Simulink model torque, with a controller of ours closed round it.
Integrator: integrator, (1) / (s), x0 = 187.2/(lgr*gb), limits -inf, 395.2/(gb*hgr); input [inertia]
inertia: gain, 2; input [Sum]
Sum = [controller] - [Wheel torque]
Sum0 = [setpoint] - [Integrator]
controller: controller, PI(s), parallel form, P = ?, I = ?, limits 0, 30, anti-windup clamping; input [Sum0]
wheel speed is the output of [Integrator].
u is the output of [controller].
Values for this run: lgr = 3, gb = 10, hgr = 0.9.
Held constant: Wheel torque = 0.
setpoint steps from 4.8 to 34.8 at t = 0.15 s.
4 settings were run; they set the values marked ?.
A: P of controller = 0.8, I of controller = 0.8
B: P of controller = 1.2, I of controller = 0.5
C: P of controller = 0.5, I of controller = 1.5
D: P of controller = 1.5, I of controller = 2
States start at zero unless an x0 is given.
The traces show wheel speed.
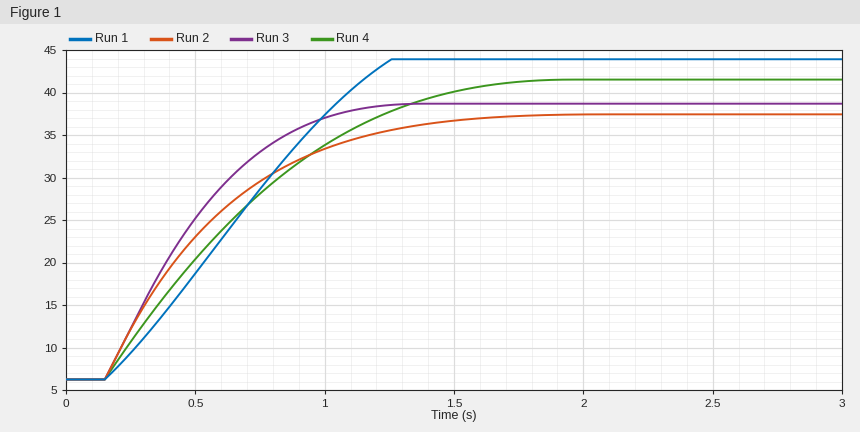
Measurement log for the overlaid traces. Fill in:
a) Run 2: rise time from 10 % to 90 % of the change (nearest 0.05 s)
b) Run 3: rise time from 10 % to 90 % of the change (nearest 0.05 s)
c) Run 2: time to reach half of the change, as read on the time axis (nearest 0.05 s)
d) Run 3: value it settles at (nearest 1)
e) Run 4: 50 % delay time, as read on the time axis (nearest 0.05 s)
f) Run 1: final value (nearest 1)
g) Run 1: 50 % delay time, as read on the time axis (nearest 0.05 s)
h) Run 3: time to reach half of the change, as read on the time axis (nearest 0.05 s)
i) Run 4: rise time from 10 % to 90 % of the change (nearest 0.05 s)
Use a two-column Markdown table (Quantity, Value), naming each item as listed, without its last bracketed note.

| Quantity | Value |
|---|---|
| Run 2: rise time from 10 % to 90 % of the change | 0.90 s |
| Run 3: rise time from 10 % to 90 % of the change | 0.65 s |
| Run 2: time to reach half of the change, as read on the time axis | 0.45 s |
| Run 3: value it settles at | 39 |
| Run 4: 50 % delay time, as read on the time axis | 0.60 s |
| Run 1: final value | 44 |
| Run 1: 50 % delay time, as read on the time axis | 0.65 s |
| Run 3: time to reach half of the change, as read on the time axis | 0.45 s |
| Run 4: rise time from 10 % to 90 % of the change | 1.05 s |
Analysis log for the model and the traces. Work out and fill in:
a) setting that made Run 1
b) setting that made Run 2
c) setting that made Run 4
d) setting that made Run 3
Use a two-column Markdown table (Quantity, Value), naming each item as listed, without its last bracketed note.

| Quantity | Value |
|---|---|
| setting that made Run 1 | C |
| setting that made Run 2 | B |
| setting that made Run 4 | A |
| setting that made Run 3 | D |
